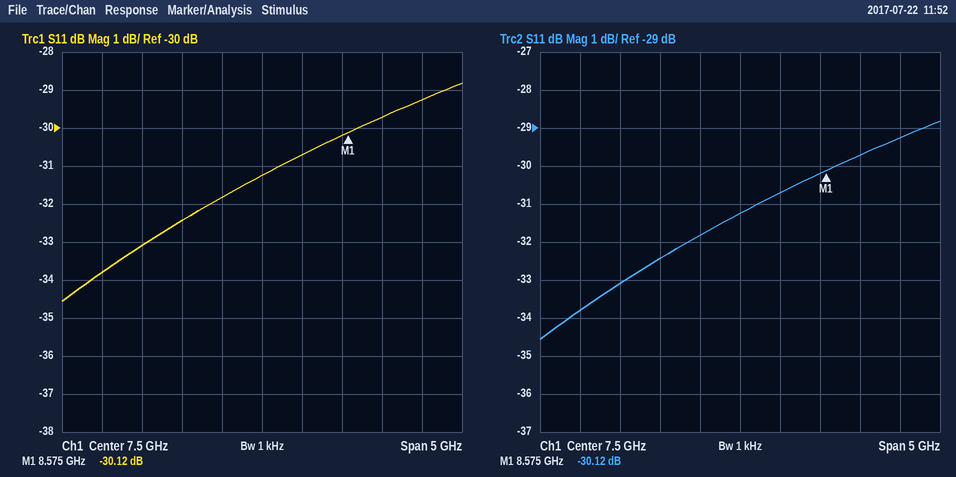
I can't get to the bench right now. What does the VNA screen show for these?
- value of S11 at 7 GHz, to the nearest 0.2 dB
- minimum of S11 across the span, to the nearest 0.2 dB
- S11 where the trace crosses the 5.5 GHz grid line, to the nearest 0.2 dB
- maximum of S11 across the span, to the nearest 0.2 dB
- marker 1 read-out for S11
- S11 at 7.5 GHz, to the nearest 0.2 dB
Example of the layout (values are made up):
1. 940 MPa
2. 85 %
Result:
1. -31.8 dB
2. -34.6 dB
3. -33.8 dB
4. -28.8 dB
5. -30.12 dB
6. -31.2 dB
